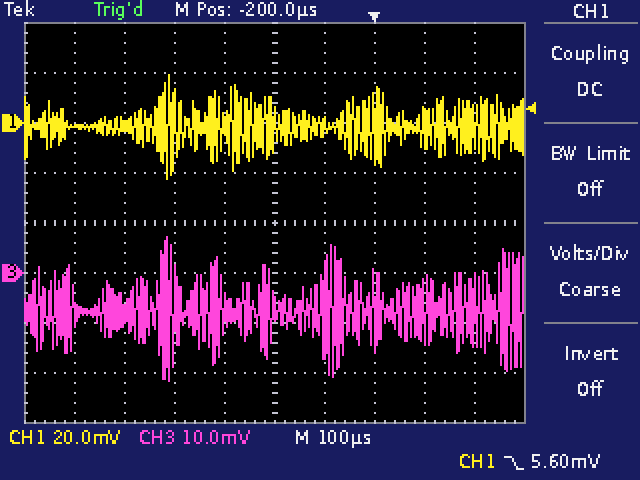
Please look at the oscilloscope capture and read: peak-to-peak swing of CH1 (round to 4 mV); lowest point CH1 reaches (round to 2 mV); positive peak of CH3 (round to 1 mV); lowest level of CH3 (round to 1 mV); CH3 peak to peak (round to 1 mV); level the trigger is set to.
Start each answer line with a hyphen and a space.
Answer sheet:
- 40 mV
- -22 mV
- 7 mV
- -22 mV
- 29 mV
- 5.60 mV
